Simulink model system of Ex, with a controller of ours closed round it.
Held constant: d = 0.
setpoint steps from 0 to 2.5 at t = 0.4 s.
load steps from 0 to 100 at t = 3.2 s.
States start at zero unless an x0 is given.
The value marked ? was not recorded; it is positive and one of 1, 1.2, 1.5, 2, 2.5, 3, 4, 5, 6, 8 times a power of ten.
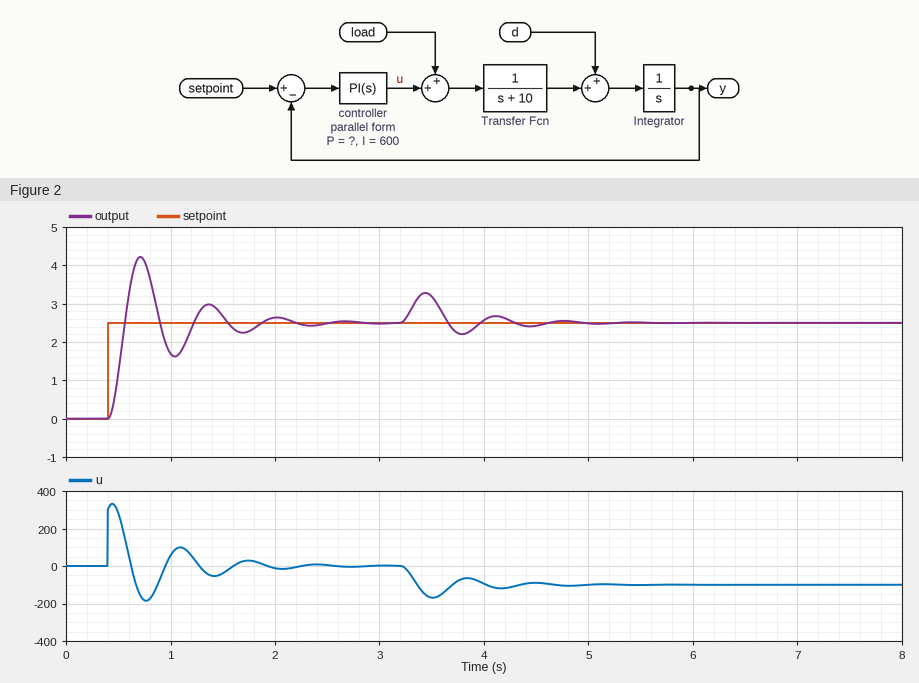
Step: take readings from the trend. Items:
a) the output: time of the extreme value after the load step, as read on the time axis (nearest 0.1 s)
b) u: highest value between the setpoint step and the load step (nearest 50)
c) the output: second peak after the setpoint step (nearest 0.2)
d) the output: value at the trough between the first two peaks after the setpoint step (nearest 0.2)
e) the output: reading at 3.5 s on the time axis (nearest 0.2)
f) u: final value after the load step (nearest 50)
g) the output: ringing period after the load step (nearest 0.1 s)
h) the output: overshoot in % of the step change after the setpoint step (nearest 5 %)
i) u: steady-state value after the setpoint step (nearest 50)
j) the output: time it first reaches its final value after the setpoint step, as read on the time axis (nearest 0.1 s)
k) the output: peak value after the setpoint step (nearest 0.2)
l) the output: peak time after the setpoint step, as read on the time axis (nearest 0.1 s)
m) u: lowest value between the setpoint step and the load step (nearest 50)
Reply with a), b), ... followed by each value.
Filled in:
a) 3.4 s
b) 350
c) 3.0
d) 1.6
e) 3.2
f) -100
g) 0.7 s
h) 70 %
i) 0
j) 0.6 s
k) 4.2
l) 0.7 s
m) -200
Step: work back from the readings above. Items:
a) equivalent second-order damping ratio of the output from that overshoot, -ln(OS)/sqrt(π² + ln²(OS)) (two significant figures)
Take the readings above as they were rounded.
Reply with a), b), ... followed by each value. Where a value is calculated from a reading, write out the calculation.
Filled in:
a) ln(0.7) = -0.357; 0.357 / sqrt(9.870 + 0.127) = 0.11
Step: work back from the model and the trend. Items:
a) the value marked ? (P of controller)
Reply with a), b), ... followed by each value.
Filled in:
a) 120
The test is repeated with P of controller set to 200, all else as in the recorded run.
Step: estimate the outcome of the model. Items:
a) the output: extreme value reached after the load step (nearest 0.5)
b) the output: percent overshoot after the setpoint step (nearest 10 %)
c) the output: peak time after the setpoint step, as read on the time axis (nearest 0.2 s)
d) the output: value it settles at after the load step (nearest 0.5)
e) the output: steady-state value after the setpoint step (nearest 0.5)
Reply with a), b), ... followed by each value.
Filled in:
a) 3.0
b) 60 %
c) 0.6 s
d) 2.5
e) 2.5
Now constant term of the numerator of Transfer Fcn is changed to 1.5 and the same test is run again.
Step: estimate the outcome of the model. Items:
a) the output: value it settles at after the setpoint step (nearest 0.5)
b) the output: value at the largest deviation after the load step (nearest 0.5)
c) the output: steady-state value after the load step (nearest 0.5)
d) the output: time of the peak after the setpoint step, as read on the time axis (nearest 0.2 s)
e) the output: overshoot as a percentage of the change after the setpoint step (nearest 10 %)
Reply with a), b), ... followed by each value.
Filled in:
a) 2.5
b) 3.5
c) 2.5
d) 0.6 s
e) 70 %
